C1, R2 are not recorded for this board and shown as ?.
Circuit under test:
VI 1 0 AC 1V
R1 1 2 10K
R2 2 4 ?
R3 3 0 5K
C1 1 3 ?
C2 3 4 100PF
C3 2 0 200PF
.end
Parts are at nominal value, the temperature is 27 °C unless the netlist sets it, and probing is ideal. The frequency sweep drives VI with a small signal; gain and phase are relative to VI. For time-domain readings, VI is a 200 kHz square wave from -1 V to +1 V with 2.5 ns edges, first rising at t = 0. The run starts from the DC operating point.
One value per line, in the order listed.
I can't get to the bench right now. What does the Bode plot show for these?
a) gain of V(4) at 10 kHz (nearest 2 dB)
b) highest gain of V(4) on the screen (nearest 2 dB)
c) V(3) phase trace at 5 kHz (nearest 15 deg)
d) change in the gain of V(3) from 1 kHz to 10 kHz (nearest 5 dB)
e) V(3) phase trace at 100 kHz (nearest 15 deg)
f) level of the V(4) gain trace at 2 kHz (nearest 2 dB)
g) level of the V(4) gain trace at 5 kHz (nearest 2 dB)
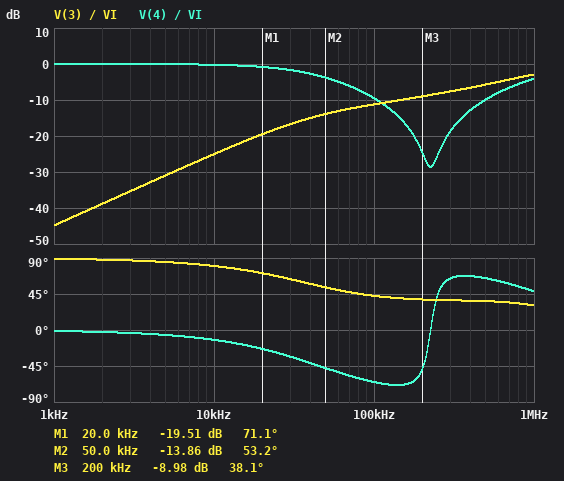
0 dB
0 dB
90 deg
20 dB
45 deg
0 dB
0 dB
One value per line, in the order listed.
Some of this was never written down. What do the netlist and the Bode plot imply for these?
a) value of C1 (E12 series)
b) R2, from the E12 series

82 pF
4.7 kΩ
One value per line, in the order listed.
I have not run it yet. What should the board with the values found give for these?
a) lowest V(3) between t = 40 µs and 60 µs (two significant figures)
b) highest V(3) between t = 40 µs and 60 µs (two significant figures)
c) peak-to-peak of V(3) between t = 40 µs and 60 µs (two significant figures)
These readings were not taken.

-1.8 V
1.8 V
3.7 V
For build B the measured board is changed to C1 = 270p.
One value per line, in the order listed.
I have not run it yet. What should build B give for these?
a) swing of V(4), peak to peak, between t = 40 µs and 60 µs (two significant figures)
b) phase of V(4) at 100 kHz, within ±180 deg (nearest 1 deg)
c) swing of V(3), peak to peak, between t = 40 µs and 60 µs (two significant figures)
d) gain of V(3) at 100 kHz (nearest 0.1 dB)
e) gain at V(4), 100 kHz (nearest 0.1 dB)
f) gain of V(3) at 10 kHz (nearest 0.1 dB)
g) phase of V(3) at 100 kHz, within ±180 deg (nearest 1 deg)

3.3 V
-42 deg
3.3 V
-4.5 dB
-11.9 dB
-18.9 dB
37 deg
